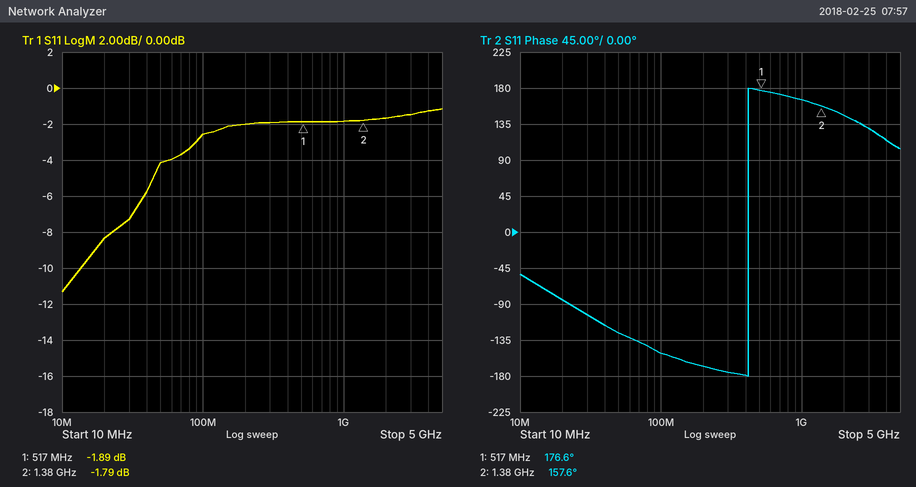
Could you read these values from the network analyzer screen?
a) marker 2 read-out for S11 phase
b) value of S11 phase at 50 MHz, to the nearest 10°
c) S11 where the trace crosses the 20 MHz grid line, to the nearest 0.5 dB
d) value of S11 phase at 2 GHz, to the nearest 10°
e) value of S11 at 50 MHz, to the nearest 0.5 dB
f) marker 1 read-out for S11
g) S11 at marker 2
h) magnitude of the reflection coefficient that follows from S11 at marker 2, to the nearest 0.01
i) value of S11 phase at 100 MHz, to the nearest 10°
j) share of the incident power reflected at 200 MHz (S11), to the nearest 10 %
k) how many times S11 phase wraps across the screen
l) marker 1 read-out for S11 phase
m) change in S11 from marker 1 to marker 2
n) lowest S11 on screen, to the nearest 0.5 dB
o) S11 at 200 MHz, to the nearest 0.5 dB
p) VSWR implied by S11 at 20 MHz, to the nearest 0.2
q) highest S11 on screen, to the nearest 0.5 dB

157.6°
-130°
-8.5 dB
150°
-4.0 dB
-1.89 dB
-1.79 dB
0.81
-150°
60 %
1
176.6°
0.10 dB
-11.5 dB
-2.0 dB
2.2
-1.0 dB
